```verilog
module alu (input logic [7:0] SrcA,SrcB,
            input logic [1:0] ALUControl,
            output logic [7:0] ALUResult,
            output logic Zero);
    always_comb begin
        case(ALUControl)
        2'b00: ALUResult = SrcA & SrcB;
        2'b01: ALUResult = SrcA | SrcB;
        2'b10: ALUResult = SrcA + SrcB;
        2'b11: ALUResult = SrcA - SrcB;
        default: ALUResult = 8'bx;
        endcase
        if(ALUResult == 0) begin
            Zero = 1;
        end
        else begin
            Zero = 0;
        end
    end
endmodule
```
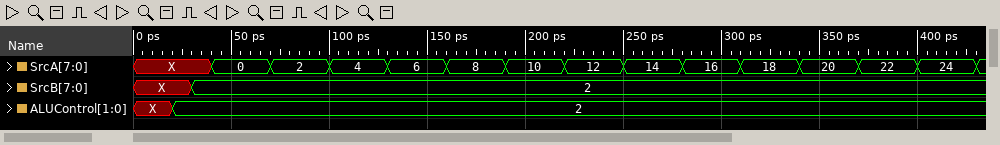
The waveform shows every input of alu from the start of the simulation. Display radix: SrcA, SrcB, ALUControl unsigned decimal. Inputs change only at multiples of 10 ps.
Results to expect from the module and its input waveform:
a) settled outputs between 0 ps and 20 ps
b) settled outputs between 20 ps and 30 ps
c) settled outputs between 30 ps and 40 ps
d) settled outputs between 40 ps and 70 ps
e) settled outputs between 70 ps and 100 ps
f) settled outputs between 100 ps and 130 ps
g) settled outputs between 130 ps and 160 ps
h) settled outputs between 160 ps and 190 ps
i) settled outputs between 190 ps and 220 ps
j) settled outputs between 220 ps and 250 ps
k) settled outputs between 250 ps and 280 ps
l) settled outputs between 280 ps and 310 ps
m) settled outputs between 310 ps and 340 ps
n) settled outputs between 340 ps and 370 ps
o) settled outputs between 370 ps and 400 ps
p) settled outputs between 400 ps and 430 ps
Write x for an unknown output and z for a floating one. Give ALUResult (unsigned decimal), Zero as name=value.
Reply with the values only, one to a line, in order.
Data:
ALUResult=x, Zero=0
ALUResult=x, Zero=0
ALUResult=x, Zero=0
ALUResult=2, Zero=0
ALUResult=4, Zero=0
ALUResult=6, Zero=0
ALUResult=8, Zero=0
ALUResult=10, Zero=0
ALUResult=12, Zero=0
ALUResult=14, Zero=0
ALUResult=16, Zero=0
ALUResult=18, Zero=0
ALUResult=20, Zero=0
ALUResult=22, Zero=0
ALUResult=24, Zero=0
ALUResult=26, Zero=0
